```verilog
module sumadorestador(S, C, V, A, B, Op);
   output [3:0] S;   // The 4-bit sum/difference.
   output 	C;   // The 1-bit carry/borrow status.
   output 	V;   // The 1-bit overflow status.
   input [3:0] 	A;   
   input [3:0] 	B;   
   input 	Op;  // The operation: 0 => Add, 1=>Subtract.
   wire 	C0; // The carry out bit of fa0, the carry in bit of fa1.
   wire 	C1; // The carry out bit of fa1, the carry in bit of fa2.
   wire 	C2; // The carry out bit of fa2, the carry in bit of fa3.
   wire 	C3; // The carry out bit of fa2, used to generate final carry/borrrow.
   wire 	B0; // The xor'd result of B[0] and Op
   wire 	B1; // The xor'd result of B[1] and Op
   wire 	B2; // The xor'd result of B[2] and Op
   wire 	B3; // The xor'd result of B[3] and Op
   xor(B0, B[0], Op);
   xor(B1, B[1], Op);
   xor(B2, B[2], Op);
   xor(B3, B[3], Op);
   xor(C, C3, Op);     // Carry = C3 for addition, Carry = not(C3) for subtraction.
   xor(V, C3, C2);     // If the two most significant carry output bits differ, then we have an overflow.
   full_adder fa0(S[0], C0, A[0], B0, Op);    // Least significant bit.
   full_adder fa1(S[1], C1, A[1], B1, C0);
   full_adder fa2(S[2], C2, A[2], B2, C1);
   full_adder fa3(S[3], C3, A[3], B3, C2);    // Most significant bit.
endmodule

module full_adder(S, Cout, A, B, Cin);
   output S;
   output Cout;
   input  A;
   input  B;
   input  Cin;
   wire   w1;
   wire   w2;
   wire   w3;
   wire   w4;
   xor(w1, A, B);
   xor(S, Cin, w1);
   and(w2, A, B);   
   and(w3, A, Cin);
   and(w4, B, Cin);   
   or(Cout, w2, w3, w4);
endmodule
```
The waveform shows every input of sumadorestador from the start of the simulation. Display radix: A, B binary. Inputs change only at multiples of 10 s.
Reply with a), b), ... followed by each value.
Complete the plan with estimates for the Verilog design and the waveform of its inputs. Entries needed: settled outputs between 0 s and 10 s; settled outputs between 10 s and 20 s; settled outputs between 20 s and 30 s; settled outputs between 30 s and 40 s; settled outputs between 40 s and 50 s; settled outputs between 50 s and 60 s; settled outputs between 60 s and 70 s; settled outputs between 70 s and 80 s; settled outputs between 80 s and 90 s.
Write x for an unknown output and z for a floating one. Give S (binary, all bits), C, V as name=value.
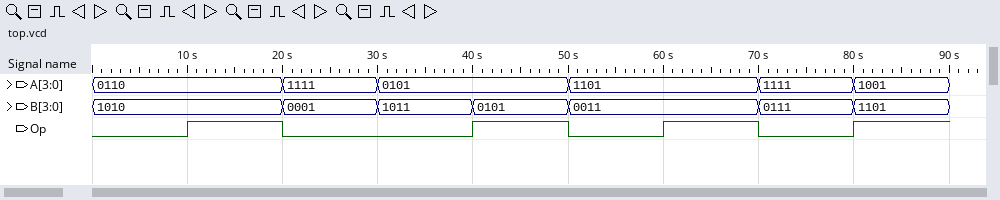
a) S=0000, C=1, V=0
b) S=1100, C=1, V=1
c) S=0000, C=1, V=0
d) S=0000, C=1, V=0
e) S=0000, C=0, V=0
f) S=0000, C=1, V=0
g) S=1010, C=0, V=0
h) S=0110, C=1, V=0
i) S=1100, C=1, V=0
